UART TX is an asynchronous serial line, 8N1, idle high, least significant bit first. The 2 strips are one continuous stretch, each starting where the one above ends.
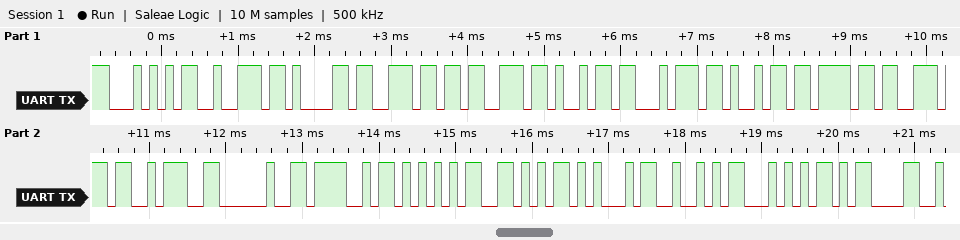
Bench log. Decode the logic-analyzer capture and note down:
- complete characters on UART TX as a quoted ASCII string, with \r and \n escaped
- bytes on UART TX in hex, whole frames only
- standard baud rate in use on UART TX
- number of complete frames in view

"Transition: OUVERT\r"
0x54 0x72 0x61 0x6E 0x73 0x69 0x74 0x69 0x6F 0x6E 0x3A 0x20 0x4F 0x55 0x56 0x45 0x52 0x54 0x0D
9600 baud
19
